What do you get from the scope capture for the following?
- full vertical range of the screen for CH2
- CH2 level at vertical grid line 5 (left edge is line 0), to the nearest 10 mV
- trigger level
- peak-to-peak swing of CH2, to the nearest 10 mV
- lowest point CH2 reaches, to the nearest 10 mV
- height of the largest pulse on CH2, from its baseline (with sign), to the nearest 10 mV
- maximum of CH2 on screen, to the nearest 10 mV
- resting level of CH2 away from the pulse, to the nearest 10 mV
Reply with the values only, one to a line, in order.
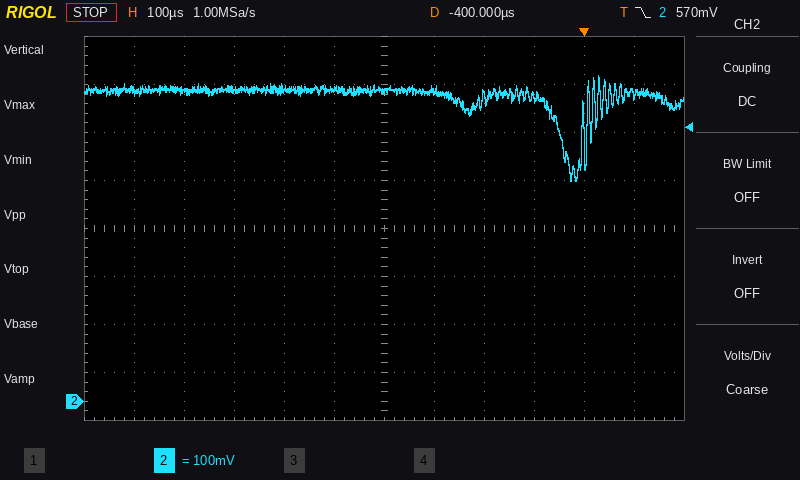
800 mV
650 mV
570 mV
220 mV
460 mV
-190 mV
680 mV
650 mV
